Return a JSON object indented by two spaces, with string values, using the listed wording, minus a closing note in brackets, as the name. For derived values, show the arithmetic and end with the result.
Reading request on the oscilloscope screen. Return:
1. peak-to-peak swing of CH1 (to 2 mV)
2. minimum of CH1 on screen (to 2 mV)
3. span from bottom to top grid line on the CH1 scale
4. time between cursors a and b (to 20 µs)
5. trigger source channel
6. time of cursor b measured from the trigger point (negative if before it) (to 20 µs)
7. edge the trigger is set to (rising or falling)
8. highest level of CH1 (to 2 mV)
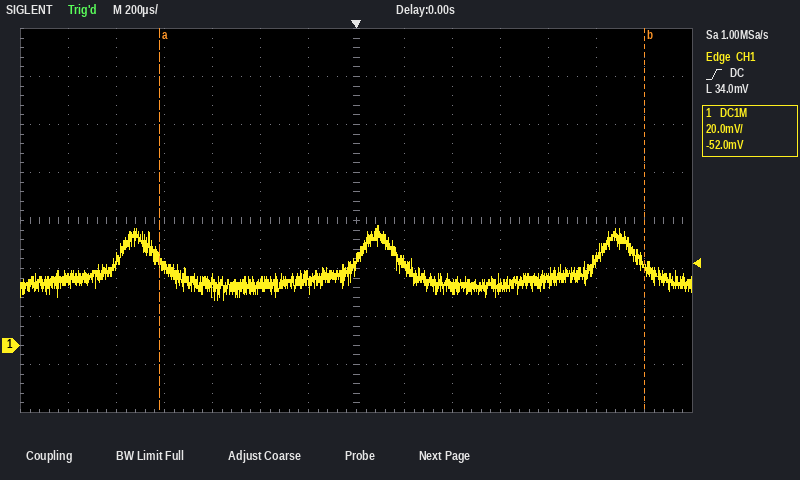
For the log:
{
  "peak-to-peak swing of CH1": "50 mV − (18 mV) = 32 mV",
  "minimum of CH1 on screen": "18 mV",
  "span from bottom to top grid line on the CH1 scale": "160 mV",
  "time between cursors a and b": "2.02 ms",
  "trigger source channel": "CH1",
  "time of cursor b measured from the trigger point (negative if before it)": "+1.20 ms",
  "edge the trigger is set to": "rising",
  "highest level of CH1": "50 mV"
}
